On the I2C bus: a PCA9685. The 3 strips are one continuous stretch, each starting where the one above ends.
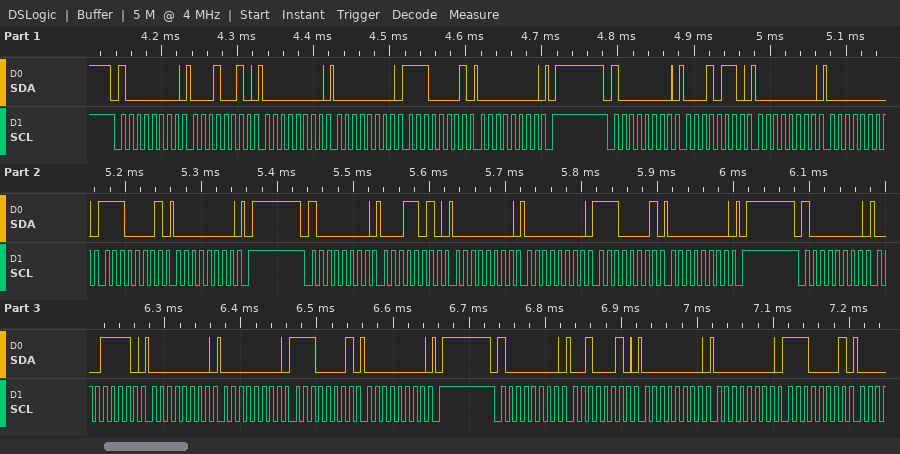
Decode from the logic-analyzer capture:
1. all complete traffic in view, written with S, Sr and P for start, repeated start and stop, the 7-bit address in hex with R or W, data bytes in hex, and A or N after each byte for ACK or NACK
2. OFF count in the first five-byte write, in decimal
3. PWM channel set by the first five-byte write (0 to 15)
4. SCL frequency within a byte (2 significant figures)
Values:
S 40W A 12 A 00 A 00 A E1 A 00 A P S 40W A 16 A 00 A 00 A E1 A 00 A P S 40W A 1A A 00 A 00 A E1 A 00 A P S 40W A 1E A 00 A 00 A E1 A 00 A P S 40W A 22 A 00 A 00 A E1 A
225
3
100 kHz
